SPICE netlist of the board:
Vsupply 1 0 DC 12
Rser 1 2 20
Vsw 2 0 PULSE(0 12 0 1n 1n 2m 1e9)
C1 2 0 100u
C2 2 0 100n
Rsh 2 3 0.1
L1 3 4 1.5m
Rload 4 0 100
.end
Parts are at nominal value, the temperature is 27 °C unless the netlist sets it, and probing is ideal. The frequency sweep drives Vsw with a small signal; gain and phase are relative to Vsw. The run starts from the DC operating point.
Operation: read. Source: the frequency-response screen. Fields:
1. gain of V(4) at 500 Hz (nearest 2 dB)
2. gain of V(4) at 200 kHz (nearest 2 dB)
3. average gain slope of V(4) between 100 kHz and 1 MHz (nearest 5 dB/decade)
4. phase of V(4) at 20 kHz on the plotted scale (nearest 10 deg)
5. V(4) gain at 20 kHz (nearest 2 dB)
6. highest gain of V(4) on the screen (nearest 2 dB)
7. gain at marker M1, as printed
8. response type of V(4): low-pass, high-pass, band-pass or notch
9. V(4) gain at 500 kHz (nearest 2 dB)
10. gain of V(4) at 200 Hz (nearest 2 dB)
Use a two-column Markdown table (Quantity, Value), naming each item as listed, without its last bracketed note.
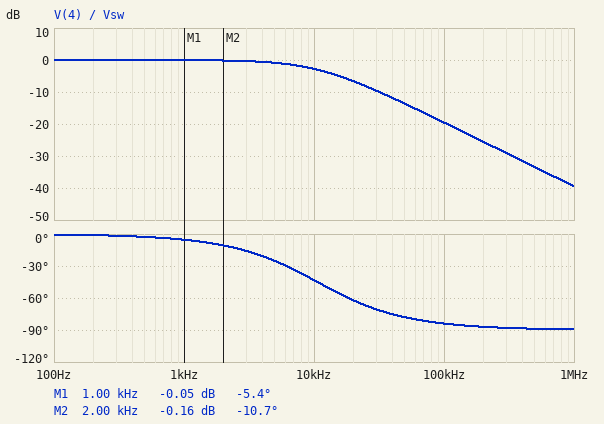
| Quantity | Value |
|---|---|
| gain of V(4) at 500 Hz | 0 dB |
| gain of V(4) at 200 kHz | -26 dB |
| average gain slope of V(4) between 100 kHz and 1 MHz | -20 dB/decade |
| phase of V(4) at 20 kHz on the plotted scale | -60 deg |
| V(4) gain at 20 kHz | -6 dB |
| highest gain of V(4) on the screen | 0 dB |
| gain at marker M1, as printed | -0.05 dB |
| response type of V(4): low-pass, high-pass, band-pass or notch | low-pass |
| V(4) gain at 500 kHz | -34 dB |
| gain of V(4) at 200 Hz | 0 dB |
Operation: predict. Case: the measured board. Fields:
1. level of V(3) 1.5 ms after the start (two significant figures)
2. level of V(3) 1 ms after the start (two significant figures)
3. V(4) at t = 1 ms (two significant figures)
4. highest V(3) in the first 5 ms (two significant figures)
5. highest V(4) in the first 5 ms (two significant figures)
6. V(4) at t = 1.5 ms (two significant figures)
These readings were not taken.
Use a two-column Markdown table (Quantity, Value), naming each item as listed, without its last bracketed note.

| Quantity | Value |
|---|---|
| level of V(3) 1.5 ms after the start | 12 V |
| level of V(3) 1 ms after the start | 12 V |
| V(4) at t = 1 ms | 12 V |
| highest V(3) in the first 5 ms | 12 V |
| highest V(4) in the first 5 ms | 12 V |
| V(4) at t = 1.5 ms | 12 V |
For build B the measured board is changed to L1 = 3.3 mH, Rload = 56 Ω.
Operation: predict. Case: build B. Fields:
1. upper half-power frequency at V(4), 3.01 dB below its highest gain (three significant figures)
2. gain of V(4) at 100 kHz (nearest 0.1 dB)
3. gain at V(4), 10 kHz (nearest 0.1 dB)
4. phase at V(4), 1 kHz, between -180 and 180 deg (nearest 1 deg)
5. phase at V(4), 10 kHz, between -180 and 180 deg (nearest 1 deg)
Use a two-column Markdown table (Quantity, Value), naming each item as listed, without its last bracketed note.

| Quantity | Value |
|---|---|
| upper half-power frequency at V(4), 3.01 dB below its highest gain | 2.71 kHz |
| gain of V(4) at 100 kHz | -31.4 dB |
| gain at V(4), 10 kHz | -11.7 dB |
| phase at V(4), 1 kHz, between -180 and 180 deg | -20 deg |
| phase at V(4), 10 kHz, between -180 and 180 deg | -75 deg |
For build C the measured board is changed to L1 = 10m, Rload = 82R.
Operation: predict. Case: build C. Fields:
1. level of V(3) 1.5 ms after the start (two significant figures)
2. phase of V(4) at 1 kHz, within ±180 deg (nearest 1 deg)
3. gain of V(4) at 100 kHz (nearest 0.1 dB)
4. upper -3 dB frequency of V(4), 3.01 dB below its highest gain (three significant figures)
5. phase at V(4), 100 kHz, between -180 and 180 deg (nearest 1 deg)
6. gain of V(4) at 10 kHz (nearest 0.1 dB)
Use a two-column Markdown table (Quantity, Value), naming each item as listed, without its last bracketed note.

| Quantity | Value |
|---|---|
| level of V(3) 1.5 ms after the start | 12 V |
| phase of V(4) at 1 kHz, within ±180 deg | -37 deg |
| gain of V(4) at 100 kHz | -37.7 dB |
| upper -3 dB frequency of V(4), 3.01 dB below its highest gain | 1.31 kHz |
| phase at V(4), 100 kHz, between -180 and 180 deg | -89 deg |
| gain of V(4) at 10 kHz | -17.8 dB |
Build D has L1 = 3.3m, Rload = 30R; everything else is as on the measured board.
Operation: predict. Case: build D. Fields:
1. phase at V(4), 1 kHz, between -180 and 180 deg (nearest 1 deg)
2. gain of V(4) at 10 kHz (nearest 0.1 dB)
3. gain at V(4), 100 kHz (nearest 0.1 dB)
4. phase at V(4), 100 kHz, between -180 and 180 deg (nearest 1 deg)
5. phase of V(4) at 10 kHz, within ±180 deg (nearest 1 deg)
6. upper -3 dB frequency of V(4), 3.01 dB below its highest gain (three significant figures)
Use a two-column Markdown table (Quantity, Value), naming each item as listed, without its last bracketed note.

| Quantity | Value |
|---|---|
| phase at V(4), 1 kHz, between -180 and 180 deg | -35 deg |
| gain of V(4) at 10 kHz | -16.9 dB |
| gain at V(4), 100 kHz | -36.8 dB |
| phase at V(4), 100 kHz, between -180 and 180 deg | -89 deg |
| phase of V(4) at 10 kHz, within ±180 deg | -82 deg |
| upper -3 dB frequency of V(4), 3.01 dB below its highest gain | 1.45 kHz |
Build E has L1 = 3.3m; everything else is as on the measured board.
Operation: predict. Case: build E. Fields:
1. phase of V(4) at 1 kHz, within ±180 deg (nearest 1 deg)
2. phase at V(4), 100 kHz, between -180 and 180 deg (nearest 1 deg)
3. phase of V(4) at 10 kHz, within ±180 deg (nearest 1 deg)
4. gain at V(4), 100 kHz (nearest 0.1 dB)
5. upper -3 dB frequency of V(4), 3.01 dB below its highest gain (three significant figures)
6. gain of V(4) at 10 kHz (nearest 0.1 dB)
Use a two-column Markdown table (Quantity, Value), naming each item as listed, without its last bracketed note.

| Quantity | Value |
|---|---|
| phase of V(4) at 1 kHz, within ±180 deg | -12 deg |
| phase at V(4), 100 kHz, between -180 and 180 deg | -87 deg |
| phase of V(4) at 10 kHz, within ±180 deg | -64 deg |
| gain at V(4), 100 kHz | -26.3 dB |
| upper -3 dB frequency of V(4), 3.01 dB below its highest gain | 4.83 kHz |
| gain of V(4) at 10 kHz | -7.2 dB |
